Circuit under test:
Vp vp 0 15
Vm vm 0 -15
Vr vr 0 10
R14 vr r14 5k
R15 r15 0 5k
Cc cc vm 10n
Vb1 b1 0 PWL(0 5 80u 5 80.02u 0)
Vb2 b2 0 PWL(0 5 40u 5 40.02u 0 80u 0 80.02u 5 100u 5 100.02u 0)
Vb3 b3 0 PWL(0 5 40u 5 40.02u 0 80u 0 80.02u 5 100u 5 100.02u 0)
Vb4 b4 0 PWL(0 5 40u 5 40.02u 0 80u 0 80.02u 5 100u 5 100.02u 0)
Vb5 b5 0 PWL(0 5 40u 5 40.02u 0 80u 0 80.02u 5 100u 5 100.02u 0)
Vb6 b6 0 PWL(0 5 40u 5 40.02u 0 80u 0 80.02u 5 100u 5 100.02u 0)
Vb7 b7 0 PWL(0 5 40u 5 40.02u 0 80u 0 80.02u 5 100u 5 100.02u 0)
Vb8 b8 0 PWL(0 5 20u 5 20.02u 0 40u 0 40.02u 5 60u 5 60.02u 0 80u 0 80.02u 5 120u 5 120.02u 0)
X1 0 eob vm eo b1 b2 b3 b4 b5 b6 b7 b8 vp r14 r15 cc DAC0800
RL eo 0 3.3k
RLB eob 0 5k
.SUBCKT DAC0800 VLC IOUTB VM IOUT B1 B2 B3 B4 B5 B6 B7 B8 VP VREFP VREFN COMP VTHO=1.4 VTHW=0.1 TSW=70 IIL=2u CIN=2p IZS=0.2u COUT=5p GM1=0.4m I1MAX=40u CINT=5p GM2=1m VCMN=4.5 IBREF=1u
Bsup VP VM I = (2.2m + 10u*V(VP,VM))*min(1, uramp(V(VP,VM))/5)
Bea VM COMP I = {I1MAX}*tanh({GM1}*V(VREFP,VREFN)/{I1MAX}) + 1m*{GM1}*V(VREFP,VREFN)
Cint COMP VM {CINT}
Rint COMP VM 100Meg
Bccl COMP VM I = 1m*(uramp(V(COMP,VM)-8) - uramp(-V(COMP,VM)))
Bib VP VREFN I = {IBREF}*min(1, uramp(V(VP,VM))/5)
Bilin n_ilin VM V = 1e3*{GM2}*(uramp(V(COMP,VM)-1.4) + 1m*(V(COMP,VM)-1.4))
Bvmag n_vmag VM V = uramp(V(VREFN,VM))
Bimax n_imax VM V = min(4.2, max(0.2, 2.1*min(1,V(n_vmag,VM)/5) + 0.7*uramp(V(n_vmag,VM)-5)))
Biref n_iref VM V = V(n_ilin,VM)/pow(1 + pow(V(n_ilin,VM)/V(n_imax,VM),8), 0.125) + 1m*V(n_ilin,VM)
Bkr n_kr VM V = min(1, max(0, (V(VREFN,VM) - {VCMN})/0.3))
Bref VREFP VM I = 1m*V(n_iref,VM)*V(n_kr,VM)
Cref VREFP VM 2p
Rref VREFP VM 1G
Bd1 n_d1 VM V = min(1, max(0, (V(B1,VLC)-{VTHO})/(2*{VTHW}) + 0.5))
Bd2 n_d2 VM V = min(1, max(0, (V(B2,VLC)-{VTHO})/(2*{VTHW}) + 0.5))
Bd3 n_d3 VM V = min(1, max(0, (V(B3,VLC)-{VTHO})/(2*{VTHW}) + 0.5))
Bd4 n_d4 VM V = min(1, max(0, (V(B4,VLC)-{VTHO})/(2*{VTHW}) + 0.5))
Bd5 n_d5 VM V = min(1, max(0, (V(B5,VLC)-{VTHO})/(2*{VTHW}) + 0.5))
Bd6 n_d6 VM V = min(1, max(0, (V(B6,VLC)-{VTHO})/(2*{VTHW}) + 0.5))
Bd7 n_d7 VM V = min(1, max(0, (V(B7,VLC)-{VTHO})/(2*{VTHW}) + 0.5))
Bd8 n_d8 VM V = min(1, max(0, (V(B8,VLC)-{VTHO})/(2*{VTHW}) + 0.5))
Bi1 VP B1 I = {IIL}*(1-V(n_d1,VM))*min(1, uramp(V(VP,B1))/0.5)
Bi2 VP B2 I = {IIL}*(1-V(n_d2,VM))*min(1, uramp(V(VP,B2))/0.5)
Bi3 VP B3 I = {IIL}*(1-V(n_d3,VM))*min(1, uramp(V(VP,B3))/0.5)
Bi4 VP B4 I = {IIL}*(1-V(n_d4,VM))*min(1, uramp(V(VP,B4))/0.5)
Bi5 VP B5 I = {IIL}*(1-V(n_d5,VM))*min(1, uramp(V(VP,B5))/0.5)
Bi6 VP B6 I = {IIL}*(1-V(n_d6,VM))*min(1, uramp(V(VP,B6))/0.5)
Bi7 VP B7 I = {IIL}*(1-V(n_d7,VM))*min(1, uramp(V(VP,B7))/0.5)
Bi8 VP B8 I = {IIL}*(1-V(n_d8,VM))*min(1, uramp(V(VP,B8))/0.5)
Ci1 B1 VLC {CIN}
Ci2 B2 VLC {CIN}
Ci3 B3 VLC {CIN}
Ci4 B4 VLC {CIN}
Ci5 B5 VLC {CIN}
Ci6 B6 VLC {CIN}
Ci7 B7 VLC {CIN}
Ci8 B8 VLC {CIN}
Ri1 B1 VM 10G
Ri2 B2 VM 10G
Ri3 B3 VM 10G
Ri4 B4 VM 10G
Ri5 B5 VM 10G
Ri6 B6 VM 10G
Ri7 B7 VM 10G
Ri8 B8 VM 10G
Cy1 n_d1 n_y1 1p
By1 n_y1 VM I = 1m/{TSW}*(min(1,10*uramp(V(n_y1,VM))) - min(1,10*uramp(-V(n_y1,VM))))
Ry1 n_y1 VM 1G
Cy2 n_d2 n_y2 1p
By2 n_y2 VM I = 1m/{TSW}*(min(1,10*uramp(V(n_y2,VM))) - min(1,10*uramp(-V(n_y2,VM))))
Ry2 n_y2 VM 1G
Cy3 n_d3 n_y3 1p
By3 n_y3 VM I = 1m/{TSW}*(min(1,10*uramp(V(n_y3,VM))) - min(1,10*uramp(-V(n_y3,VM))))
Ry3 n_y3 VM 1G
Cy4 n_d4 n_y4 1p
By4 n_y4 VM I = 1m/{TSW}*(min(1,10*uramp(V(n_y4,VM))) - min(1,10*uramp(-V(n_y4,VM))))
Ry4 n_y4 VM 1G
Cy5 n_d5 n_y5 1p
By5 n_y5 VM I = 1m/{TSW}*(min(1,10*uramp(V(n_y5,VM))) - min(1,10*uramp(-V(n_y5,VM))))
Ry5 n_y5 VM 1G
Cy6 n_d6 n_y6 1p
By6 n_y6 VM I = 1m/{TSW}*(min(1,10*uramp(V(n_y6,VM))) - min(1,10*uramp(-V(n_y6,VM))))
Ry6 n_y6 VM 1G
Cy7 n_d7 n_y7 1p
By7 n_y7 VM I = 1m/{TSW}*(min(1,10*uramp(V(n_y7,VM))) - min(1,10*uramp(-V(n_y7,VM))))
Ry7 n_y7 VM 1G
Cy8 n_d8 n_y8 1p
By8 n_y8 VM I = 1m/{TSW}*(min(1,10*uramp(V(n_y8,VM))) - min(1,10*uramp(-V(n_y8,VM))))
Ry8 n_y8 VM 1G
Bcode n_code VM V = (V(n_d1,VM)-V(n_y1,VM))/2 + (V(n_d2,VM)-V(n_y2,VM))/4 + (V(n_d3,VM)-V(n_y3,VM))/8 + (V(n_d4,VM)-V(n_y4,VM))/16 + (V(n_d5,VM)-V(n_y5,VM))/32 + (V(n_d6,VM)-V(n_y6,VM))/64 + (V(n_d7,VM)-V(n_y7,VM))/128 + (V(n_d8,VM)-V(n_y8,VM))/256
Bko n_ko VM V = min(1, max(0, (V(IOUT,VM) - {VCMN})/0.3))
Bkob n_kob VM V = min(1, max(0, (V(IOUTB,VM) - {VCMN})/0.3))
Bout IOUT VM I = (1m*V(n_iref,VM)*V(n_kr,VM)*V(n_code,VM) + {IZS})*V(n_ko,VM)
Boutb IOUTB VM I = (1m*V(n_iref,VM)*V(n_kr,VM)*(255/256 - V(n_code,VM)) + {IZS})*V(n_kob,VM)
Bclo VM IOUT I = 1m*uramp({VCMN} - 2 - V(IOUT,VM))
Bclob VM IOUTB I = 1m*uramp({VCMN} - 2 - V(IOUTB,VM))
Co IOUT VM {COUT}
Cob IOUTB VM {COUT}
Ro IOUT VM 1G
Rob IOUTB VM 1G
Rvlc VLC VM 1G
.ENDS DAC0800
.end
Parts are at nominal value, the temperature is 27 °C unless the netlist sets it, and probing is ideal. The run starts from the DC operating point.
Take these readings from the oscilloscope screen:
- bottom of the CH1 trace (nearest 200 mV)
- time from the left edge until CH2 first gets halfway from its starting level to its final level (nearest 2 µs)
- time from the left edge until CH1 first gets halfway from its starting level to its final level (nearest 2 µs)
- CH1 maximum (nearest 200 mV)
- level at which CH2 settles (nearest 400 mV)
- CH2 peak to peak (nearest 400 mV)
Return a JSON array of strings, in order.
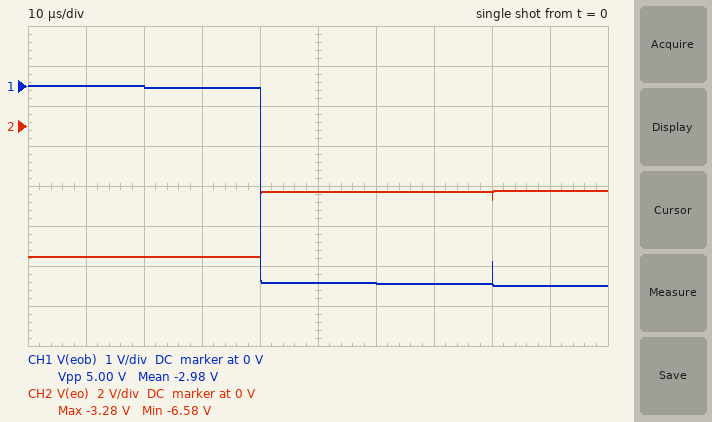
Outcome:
["-5.0 V", "40 µs", "40 µs", "0 V", "-3.2 V", "3.2 V"]
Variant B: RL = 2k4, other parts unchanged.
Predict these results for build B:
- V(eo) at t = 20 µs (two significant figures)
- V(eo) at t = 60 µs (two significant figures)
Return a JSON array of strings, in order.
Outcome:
["-4.8 V", "-2.4 V"]
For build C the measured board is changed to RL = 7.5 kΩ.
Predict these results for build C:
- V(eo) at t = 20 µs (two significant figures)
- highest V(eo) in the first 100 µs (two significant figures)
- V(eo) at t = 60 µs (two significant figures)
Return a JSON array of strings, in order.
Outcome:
["-10 V", "-7.4 V", "-7.6 V"]
